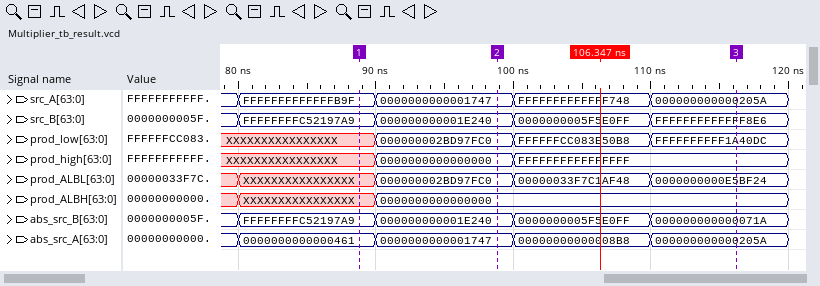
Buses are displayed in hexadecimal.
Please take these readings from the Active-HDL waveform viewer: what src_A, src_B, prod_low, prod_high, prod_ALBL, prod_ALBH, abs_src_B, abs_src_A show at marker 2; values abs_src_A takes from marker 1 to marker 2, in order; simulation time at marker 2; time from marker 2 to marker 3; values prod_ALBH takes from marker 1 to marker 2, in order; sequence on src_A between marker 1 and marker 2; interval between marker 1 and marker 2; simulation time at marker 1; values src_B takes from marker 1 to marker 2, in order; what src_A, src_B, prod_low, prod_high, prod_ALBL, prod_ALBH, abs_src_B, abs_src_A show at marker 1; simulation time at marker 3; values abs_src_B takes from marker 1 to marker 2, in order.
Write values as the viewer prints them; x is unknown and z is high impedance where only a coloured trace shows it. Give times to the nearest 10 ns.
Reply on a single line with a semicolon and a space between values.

src_A=0000000000001747, src_B=000000000001E240, prod_low=000000002BD97FC0, prod_high=0000000000000000, prod_ALBL=000000002BD97FC0, prod_ALBH=0000000000000000, abs_src_B=000000000001E240, abs_src_A=0000000000001747; 0000000000000461, 0000000000001747; 100 ns; 20 ns; XXXXXXXXXXXXXXXX, 0000000000000000; FFFFFFFFFFFFFB9F, 0000000000001747; 10 ns; 90 ns; FFFFFFFFC52197A9, 000000000001E240; src_A=FFFFFFFFFFFFFB9F, src_B=FFFFFFFFC52197A9, prod_low=XXXXXXXXXXXXXXXX, prod_high=XXXXXXXXXXXXXXXX, prod_ALBL=XXXXXXXXXXXXXXXX, prod_ALBH=XXXXXXXXXXXXXXXX, abs_src_B=FFFFFFFFC52197A9, abs_src_A=0000000000000461; 120 ns; FFFFFFFFC52197A9, 000000000001E240
